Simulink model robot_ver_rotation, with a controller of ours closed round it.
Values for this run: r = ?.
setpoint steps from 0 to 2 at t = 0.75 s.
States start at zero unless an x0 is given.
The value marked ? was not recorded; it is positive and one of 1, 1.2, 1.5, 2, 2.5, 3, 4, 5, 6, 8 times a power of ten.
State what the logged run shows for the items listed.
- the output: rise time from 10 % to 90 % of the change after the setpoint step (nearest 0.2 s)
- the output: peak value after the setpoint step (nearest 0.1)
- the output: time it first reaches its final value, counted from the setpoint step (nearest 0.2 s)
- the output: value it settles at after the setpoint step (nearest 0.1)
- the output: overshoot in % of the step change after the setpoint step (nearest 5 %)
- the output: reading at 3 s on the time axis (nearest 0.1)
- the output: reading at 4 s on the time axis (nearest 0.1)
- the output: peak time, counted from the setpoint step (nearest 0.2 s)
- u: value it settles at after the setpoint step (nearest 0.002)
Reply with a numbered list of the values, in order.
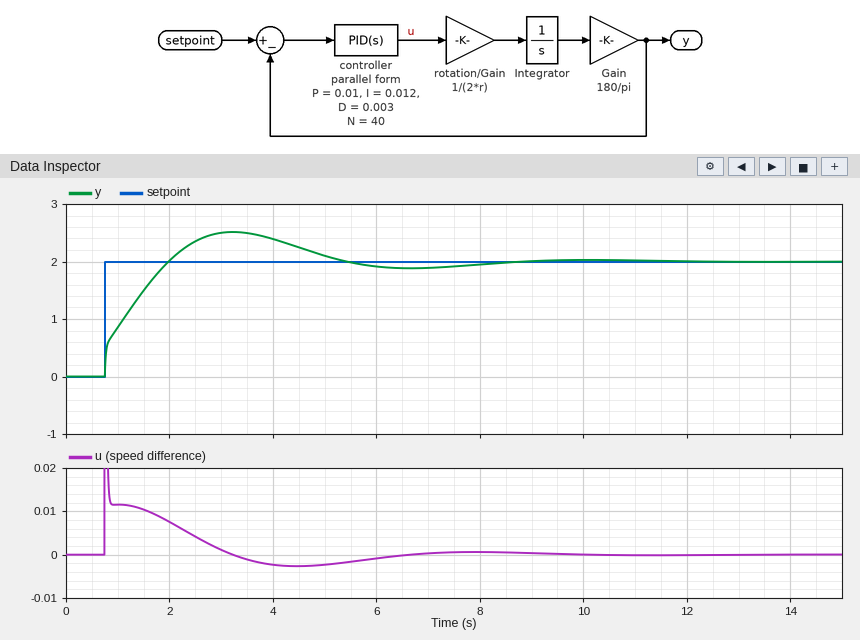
1. 1.0 s
2. 2.5
3. 1.2 s
4. 2.0
5. 25 %
6. 2.5
7. 2.4
8. 2.4 s
9. 0.000
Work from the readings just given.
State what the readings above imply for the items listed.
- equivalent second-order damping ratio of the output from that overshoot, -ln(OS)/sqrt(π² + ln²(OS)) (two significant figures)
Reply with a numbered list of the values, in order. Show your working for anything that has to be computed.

1. ln(0.25) = -1.386; 1.386 / sqrt(9.870 + 1.922) = 0.40
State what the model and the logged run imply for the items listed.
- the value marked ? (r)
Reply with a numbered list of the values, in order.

1. 0.25
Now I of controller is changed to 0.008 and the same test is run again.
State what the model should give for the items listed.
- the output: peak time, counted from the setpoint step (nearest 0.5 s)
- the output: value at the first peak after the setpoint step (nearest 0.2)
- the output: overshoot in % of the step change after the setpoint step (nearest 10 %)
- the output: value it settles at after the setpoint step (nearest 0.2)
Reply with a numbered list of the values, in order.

1. 3.0 s
2. 2.4
3. 20 %
4. 2.0
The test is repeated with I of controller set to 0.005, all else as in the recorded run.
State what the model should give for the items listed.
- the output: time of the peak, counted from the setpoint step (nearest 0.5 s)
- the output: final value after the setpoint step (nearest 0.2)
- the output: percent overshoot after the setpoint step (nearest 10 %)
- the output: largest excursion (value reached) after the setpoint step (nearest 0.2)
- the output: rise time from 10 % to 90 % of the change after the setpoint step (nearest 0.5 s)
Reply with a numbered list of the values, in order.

1. 3.5 s
2. 2.0
3. 20 %
4. 2.4
5. 1.5 s
